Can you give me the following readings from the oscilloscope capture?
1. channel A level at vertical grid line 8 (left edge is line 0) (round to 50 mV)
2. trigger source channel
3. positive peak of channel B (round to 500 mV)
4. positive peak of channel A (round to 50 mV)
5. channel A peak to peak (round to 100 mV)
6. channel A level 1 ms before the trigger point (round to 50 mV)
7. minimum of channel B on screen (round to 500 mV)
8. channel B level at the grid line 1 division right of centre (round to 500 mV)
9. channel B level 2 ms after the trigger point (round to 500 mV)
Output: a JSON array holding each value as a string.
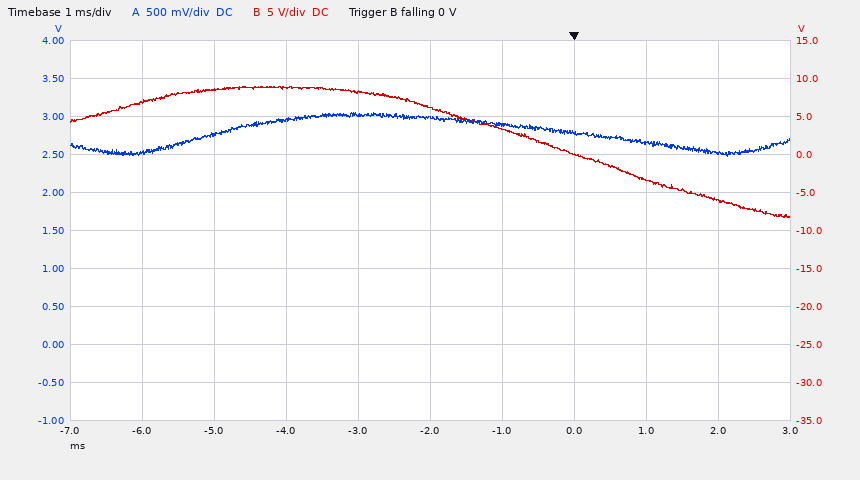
["2.65 V", "channel B", "9.0 V", "3.05 V", "600 mV", "2.90 V", "-8.5 V", "3.5 V", "-6.0 V"]
